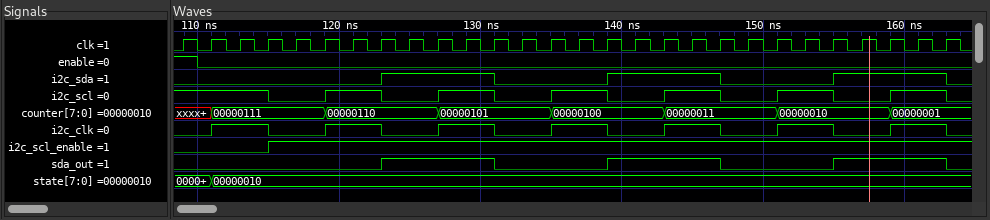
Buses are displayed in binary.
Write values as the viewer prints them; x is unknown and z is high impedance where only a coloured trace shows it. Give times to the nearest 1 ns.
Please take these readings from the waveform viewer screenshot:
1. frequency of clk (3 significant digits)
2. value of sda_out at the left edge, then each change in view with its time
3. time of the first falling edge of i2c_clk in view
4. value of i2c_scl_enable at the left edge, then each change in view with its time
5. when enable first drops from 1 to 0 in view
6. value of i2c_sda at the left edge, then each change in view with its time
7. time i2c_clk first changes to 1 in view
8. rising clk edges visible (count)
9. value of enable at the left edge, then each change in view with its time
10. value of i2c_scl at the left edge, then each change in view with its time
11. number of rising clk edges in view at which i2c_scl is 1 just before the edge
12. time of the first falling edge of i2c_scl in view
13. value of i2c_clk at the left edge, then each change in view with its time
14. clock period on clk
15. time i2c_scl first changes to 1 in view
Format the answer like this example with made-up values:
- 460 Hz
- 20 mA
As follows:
- 500 MHz
- 0, 1 at 123 ns, 0 at 131 ns, 1 at 139 ns, 0 at 147 ns, 1 at 155 ns, 0 at 163 ns
- 115 ns
- 0, 1 at 115 ns
- 110 ns
- 0, 1 at 123 ns, 0 at 131 ns, 1 at 139 ns, 0 at 147 ns, 1 at 155 ns, 0 at 163 ns
- 111 ns
- 28
- 1, 0 at 110 ns
- 1, 0 at 115 ns, 1 at 119 ns, 0 at 123 ns, 1 at 127 ns, 0 at 131 ns, 1 at 135 ns, 0 at 139 ns, 1 at 143 ns, 0 at 147 ns, 1 at 151 ns, 0 at 155 ns, 1 at 159 ns, 0 at 163 ns
- 16
- 115 ns
- 0, 1 at 111 ns, 0 at 115 ns, 1 at 119 ns, 0 at 123 ns, 1 at 127 ns, 0 at 131 ns, 1 at 135 ns, 0 at 139 ns, 1 at 143 ns, 0 at 147 ns, 1 at 151 ns, 0 at 155 ns, 1 at 159 ns, 0 at 163 ns
- 2 ns
- 119 ns
